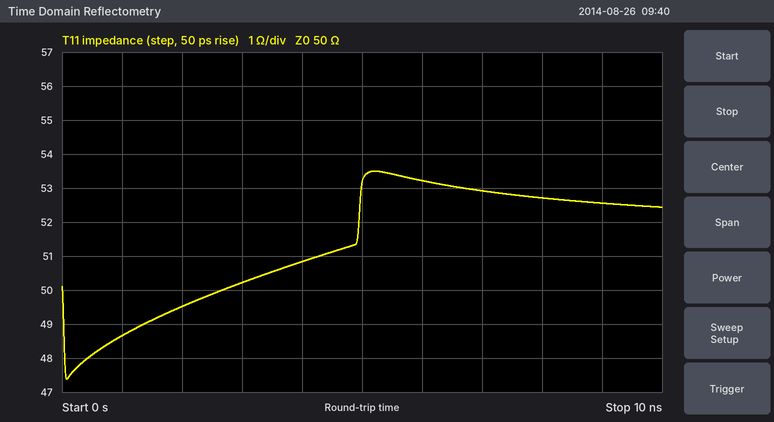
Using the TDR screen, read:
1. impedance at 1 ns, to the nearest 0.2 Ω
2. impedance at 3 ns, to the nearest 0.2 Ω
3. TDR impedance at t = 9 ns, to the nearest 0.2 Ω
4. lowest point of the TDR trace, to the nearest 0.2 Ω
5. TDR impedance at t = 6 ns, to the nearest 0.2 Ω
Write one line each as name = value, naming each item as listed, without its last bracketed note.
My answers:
impedance at 1 ns, to the nearest 0.2 Ω = 48.6 Ω
impedance at 3 ns, to the nearest 0.2 Ω = 50.2 Ω
TDR impedance at t = 9 ns, to the nearest 0.2 Ω = 52.6 Ω
lowest point of the TDR trace, to the nearest 0.2 Ω = 47.4 Ω
TDR impedance at t = 6 ns, to the nearest 0.2 Ω = 53.2 Ω
